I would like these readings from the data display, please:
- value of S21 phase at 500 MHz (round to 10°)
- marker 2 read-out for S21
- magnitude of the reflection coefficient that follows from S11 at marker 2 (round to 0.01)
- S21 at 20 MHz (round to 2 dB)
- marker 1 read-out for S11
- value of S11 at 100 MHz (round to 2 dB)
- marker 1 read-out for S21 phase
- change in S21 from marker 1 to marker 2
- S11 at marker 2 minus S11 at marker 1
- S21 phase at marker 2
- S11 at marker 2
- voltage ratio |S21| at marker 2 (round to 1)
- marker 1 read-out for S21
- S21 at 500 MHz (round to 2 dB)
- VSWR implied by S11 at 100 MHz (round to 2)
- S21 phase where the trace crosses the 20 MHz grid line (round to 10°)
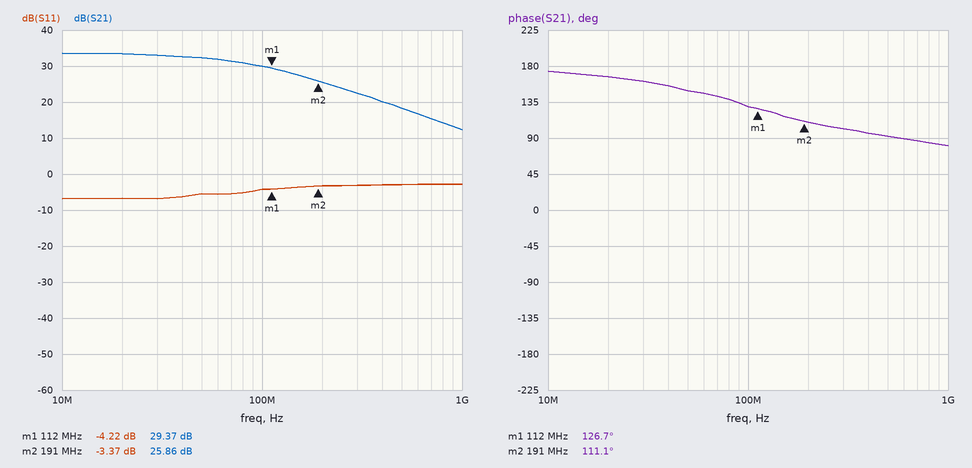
90°
25.86 dB
0.68
34 dB
-4.22 dB
-4 dB
126.7°
-3.51 dB
0.85 dB
111.1°
-3.37 dB
20
29.37 dB
18 dB
4
170°
